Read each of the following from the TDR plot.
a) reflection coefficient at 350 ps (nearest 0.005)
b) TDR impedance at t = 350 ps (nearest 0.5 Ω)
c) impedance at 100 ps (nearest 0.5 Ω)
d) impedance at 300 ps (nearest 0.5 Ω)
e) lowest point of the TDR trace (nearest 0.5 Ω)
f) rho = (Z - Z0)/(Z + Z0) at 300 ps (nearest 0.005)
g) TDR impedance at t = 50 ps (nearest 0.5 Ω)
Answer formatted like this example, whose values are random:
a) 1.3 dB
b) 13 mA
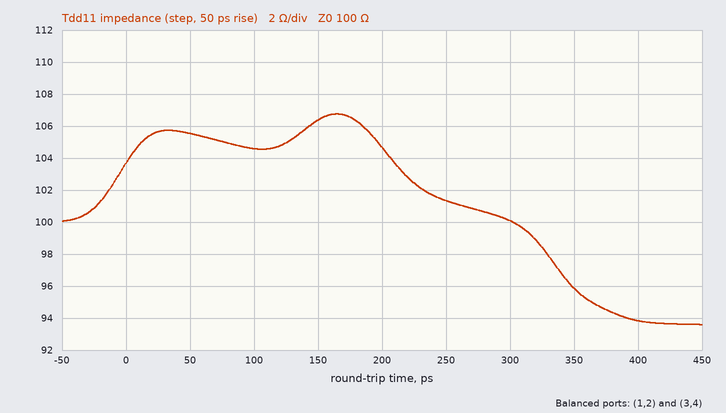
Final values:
a) -0.020
b) 96.0 Ω
c) 104.5 Ω
d) 100.0 Ω
e) 93.5 Ω
f) 0.000
g) 105.5 Ω
